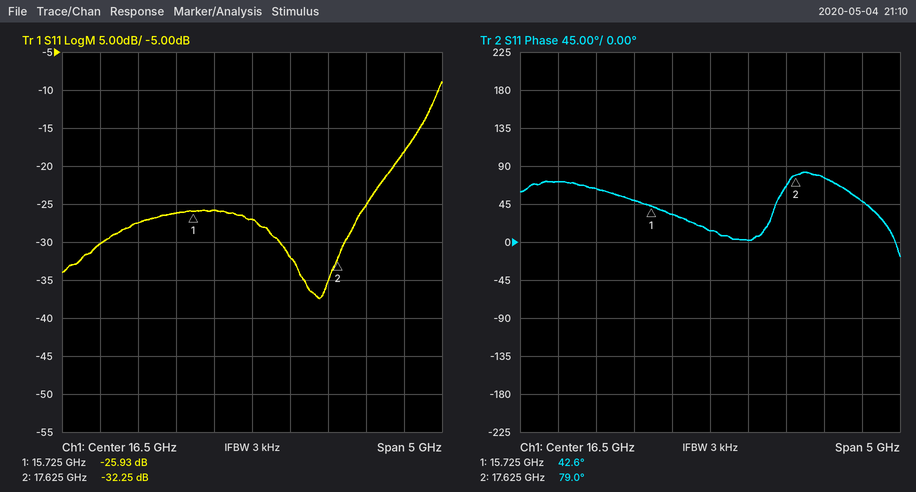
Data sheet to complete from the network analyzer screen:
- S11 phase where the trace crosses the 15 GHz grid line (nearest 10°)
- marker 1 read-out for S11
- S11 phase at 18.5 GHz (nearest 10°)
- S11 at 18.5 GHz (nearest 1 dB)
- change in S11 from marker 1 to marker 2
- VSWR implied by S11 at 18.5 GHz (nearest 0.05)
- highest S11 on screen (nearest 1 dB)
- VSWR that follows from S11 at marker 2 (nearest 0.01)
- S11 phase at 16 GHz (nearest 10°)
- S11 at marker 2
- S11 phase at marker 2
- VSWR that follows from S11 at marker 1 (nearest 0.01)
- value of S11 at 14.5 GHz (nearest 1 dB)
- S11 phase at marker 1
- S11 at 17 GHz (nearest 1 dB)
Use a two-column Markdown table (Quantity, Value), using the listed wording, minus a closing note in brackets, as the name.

| Quantity | Value |
|---|---|
| S11 phase where the trace crosses the 15 GHz grid line | 60° |
| marker 1 read-out for S11 | -25.93 dB |
| S11 phase at 18.5 GHz | 50° |
| S11 at 18.5 GHz | -18 dB |
| change in S11 from marker 1 to marker 2 | -6.32 dB |
| VSWR implied by S11 at 18.5 GHz | 1.30 |
| highest S11 on screen | -9 dB |
| VSWR that follows from S11 at marker 2 | 1.05 |
| S11 phase at 16 GHz | 30° |
| S11 at marker 2 | -32.25 dB |
| S11 phase at marker 2 | 79.0° |
| VSWR that follows from S11 at marker 1 | 1.11 |
| value of S11 at 14.5 GHz | -30 dB |
| S11 phase at marker 1 | 42.6° |
| S11 at 17 GHz | -32 dB |
